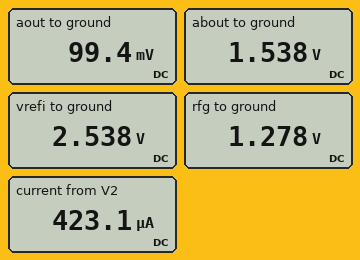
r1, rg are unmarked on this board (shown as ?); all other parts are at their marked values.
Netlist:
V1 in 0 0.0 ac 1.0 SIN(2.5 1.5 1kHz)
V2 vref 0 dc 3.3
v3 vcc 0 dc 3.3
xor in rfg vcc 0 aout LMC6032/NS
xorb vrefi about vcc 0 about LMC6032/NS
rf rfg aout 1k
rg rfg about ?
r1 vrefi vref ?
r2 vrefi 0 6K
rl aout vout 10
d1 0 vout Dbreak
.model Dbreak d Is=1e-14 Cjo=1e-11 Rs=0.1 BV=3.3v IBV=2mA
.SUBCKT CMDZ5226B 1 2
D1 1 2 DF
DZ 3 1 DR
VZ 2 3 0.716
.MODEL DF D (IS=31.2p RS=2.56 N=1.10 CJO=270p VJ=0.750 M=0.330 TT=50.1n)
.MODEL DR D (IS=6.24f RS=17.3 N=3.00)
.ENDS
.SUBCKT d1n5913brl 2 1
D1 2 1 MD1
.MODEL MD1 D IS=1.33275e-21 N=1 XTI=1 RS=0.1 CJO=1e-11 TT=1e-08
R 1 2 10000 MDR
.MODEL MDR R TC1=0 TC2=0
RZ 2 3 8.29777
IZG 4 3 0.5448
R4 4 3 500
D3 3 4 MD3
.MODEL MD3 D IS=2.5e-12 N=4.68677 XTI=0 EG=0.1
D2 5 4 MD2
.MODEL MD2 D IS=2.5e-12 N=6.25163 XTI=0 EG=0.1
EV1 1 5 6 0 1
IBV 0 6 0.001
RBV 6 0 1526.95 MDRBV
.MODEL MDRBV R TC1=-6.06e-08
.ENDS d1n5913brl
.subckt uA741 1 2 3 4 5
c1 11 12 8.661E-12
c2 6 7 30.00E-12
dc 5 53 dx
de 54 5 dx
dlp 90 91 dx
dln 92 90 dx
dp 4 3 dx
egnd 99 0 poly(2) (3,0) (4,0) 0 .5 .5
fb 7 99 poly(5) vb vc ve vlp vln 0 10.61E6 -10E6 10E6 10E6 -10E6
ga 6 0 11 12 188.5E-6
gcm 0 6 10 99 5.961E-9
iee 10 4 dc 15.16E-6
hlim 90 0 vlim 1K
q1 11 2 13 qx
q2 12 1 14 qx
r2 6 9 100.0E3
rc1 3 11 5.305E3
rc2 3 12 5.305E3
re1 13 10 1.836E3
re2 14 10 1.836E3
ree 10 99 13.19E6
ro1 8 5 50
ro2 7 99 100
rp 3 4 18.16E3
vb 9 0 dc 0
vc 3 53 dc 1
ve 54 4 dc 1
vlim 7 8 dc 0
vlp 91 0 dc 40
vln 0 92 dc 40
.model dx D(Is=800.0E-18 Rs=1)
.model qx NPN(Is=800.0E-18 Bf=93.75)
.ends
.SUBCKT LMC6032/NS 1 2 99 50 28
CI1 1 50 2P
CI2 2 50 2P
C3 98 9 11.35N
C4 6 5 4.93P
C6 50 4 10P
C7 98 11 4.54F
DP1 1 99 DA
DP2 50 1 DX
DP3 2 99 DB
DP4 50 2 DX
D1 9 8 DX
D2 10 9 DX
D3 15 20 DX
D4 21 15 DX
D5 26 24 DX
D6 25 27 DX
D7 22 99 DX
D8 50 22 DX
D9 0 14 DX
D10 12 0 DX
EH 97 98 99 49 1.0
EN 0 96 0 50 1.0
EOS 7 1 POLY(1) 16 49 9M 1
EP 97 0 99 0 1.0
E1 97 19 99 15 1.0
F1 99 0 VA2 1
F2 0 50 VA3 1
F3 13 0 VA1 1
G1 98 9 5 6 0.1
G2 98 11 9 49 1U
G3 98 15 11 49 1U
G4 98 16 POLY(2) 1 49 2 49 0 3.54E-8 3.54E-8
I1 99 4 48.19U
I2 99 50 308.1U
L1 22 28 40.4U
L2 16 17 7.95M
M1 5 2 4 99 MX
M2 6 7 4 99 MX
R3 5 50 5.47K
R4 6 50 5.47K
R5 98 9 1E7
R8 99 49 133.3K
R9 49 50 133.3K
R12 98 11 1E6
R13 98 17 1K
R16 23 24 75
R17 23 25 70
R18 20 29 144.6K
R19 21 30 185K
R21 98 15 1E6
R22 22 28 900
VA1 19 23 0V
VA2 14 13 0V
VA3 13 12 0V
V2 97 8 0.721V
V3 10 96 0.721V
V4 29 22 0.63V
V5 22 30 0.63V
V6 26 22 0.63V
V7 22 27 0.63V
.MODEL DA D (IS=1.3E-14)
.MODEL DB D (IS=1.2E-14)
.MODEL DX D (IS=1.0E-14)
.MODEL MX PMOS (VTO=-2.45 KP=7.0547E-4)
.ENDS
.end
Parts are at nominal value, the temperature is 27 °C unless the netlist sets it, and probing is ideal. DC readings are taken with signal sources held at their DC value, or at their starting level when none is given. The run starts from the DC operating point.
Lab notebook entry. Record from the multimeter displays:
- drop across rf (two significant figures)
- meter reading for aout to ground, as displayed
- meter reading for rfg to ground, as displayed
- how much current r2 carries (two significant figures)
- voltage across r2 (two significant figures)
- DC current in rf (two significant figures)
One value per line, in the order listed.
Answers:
1.2 V
99.4 mV
1.278 V
420 µA
2.5 V
1.2 mA
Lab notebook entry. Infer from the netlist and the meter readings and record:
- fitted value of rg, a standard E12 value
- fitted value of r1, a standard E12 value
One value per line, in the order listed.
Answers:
220 Ω
1.8 kΩ
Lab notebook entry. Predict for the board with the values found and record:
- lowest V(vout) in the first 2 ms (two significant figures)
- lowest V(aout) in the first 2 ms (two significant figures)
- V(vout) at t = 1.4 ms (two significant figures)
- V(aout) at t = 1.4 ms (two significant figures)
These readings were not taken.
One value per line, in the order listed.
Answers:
100 mV
100 mV
650 mV
650 mV
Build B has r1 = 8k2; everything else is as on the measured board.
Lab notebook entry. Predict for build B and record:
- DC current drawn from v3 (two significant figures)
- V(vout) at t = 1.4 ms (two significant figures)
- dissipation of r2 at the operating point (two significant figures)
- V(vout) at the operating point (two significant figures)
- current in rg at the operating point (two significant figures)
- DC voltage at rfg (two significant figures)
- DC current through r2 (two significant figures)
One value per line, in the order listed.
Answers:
1.8 mA
1.4 V
320 µW
90 mV
1.1 mA
1.2 V
230 µA
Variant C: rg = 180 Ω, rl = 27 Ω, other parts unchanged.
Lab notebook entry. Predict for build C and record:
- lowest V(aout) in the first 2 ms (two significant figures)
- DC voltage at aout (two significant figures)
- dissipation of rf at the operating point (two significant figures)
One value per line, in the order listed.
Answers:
110 mV
100 mV
1.5 mW
